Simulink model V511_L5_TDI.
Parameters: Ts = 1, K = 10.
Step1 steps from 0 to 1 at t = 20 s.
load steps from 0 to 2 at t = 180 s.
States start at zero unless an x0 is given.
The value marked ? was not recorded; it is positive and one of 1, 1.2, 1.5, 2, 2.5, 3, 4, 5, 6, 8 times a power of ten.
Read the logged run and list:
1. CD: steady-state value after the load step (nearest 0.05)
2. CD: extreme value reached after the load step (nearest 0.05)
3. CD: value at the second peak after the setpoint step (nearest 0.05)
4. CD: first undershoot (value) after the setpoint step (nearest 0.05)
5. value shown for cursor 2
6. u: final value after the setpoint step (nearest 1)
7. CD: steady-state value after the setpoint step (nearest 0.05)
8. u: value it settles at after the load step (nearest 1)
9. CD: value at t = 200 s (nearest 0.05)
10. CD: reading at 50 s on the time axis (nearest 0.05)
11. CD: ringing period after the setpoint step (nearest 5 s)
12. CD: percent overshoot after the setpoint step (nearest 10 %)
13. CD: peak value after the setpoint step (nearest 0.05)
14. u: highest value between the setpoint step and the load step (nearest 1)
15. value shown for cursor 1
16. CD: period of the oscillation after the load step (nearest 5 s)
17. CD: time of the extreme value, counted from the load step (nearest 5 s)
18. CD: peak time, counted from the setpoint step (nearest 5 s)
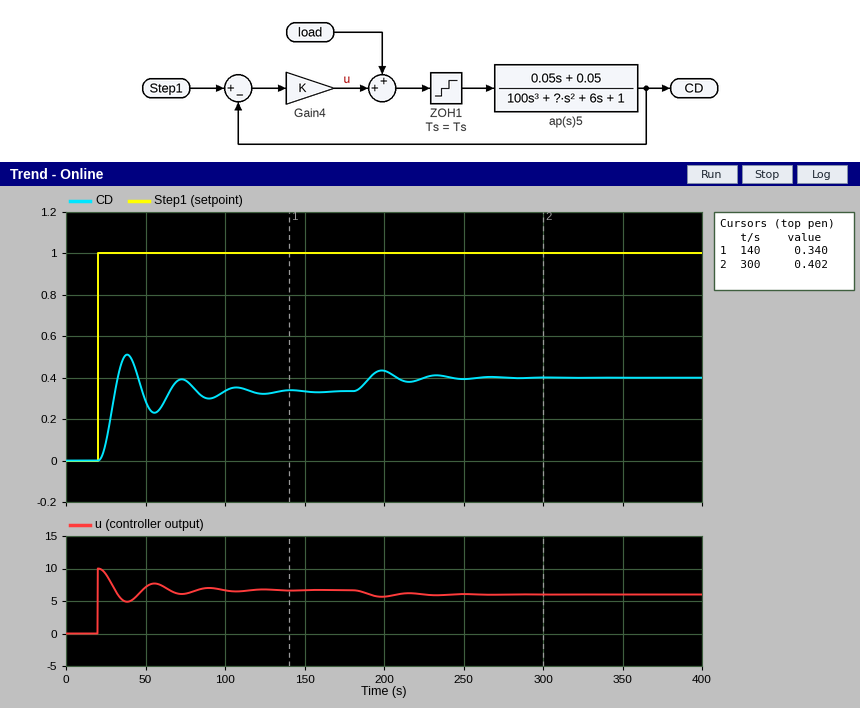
0.40
0.45
0.40
0.25
0.402
7
0.35
6
0.45
0.30
35 s
50 %
0.50
10
0.340
35 s
20 s
20 s
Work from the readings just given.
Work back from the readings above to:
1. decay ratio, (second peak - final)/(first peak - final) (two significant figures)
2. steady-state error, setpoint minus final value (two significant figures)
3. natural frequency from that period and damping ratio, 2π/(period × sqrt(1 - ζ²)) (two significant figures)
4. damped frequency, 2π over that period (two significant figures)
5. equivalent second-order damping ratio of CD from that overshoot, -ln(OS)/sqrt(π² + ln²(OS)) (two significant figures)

0.33
0.65
0.18 rad/s
0.18 rad/s
0.22
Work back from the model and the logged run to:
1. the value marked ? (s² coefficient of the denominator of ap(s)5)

50
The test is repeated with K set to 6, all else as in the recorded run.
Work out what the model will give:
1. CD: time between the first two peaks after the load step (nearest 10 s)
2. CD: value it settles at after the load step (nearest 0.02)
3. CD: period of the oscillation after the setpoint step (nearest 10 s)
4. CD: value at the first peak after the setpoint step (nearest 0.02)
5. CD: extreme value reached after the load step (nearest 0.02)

40 s
0.30
40 s
0.34
0.34
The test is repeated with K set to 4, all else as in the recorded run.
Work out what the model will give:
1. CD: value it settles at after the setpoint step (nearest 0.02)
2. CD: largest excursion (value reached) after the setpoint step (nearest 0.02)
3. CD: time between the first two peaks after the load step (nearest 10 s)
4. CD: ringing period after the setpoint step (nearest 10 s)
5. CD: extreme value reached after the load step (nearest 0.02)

0.16
0.24
40 s
40 s
0.28
